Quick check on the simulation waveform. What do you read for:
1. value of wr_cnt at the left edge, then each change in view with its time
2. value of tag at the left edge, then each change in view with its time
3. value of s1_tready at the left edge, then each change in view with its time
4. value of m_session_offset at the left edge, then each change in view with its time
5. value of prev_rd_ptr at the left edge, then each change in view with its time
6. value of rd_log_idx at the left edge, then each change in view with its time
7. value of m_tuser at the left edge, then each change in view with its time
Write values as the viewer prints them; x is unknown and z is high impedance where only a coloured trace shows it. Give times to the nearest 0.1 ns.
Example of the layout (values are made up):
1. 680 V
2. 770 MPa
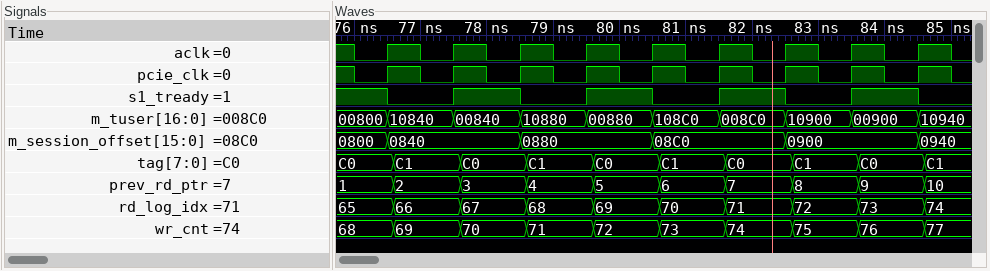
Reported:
1. 68, 69 at 76.6 ns, 70 at 77.6 ns, 71 at 78.6 ns, 72 at 79.6 ns, 73 at 80.6 ns, 74 at 81.6 ns, 75 at 82.6 ns, 76 at 83.6 ns, 77 at 84.6 ns
2. C0, C1 at 76.6 ns, C0 at 77.6 ns, C1 at 78.6 ns, C0 at 79.6 ns, C1 at 80.6 ns, C0 at 81.6 ns, C1 at 82.6 ns, C0 at 83.6 ns, C1 at 84.6 ns
3. 1, 0 at 76.5 ns, 1 at 77.5 ns, 0 at 78.5 ns, 1 at 79.5 ns, 0 at 80.5 ns, 1 at 81.5 ns, 0 at 82.5 ns, 1 at 83.5 ns, 0 at 84.5 ns
4. 0800, 0840 at 76.5 ns, 0880 at 78.5 ns, 08C0 at 80.5 ns, 0900 at 82.5 ns, 0940 at 84.5 ns
5. 1, 2 at 76.6 ns, 3 at 77.6 ns, 4 at 78.6 ns, 5 at 79.6 ns, 6 at 80.6 ns, 7 at 81.6 ns, 8 at 82.6 ns, 9 at 83.6 ns, 10 at 84.6 ns
6. 65, 66 at 76.6 ns, 67 at 77.6 ns, 68 at 78.6 ns, 69 at 79.6 ns, 70 at 80.6 ns, 71 at 81.6 ns, 72 at 82.6 ns, 73 at 83.6 ns, 74 at 84.6 ns
7. 00800, 10840 at 76.5 ns, 00840 at 77.5 ns, 10880 at 78.5 ns, 00880 at 79.5 ns, 108C0 at 80.5 ns, 008C0 at 81.5 ns, 10900 at 82.5 ns, 00900 at 83.5 ns, 10940 at 84.5 ns
